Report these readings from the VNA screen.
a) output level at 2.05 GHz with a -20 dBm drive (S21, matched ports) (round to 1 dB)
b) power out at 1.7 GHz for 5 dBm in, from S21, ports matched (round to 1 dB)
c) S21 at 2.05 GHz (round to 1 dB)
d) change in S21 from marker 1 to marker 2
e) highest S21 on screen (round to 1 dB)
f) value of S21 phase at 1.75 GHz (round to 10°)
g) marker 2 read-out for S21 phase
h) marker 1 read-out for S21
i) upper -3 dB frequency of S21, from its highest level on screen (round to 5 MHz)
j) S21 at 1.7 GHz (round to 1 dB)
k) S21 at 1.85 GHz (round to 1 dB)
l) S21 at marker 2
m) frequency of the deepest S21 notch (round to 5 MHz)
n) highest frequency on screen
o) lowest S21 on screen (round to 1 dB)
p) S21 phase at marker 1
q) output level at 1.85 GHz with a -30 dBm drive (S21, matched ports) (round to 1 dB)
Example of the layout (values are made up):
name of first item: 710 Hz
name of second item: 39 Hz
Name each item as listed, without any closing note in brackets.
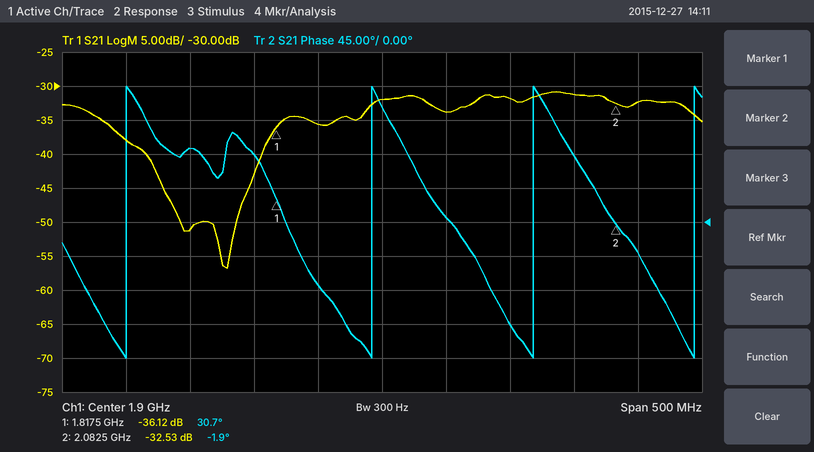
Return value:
output level at 2.05 GHz with a -20 dBm drive (S21, matched ports): -51 dBm
power out at 1.7 GHz for 5 dBm in, from S21, ports matched: -33 dBm
S21 at 2.05 GHz: -31 dB
change in S21 from marker 1 to marker 2: 3.59 dB
highest S21 on screen: -31 dB
value of S21 phase at 1.75 GHz: 100°
marker 2 read-out for S21 phase: -1.9°
marker 1 read-out for S21: -36.12 dB
upper -3 dB frequency of S21, from its highest level on screen: 2.140 GHz
S21 at 1.7 GHz: -38 dB
S21 at 1.85 GHz: -36 dB
S21 at marker 2: -32.53 dB
frequency of the deepest S21 notch: 1.780 GHz
highest frequency on screen: 2.15 GHz
lowest S21 on screen: -57 dB
S21 phase at marker 1: 30.7°
output level at 1.85 GHz with a -30 dBm drive (S21, matched ports): -66 dBm
